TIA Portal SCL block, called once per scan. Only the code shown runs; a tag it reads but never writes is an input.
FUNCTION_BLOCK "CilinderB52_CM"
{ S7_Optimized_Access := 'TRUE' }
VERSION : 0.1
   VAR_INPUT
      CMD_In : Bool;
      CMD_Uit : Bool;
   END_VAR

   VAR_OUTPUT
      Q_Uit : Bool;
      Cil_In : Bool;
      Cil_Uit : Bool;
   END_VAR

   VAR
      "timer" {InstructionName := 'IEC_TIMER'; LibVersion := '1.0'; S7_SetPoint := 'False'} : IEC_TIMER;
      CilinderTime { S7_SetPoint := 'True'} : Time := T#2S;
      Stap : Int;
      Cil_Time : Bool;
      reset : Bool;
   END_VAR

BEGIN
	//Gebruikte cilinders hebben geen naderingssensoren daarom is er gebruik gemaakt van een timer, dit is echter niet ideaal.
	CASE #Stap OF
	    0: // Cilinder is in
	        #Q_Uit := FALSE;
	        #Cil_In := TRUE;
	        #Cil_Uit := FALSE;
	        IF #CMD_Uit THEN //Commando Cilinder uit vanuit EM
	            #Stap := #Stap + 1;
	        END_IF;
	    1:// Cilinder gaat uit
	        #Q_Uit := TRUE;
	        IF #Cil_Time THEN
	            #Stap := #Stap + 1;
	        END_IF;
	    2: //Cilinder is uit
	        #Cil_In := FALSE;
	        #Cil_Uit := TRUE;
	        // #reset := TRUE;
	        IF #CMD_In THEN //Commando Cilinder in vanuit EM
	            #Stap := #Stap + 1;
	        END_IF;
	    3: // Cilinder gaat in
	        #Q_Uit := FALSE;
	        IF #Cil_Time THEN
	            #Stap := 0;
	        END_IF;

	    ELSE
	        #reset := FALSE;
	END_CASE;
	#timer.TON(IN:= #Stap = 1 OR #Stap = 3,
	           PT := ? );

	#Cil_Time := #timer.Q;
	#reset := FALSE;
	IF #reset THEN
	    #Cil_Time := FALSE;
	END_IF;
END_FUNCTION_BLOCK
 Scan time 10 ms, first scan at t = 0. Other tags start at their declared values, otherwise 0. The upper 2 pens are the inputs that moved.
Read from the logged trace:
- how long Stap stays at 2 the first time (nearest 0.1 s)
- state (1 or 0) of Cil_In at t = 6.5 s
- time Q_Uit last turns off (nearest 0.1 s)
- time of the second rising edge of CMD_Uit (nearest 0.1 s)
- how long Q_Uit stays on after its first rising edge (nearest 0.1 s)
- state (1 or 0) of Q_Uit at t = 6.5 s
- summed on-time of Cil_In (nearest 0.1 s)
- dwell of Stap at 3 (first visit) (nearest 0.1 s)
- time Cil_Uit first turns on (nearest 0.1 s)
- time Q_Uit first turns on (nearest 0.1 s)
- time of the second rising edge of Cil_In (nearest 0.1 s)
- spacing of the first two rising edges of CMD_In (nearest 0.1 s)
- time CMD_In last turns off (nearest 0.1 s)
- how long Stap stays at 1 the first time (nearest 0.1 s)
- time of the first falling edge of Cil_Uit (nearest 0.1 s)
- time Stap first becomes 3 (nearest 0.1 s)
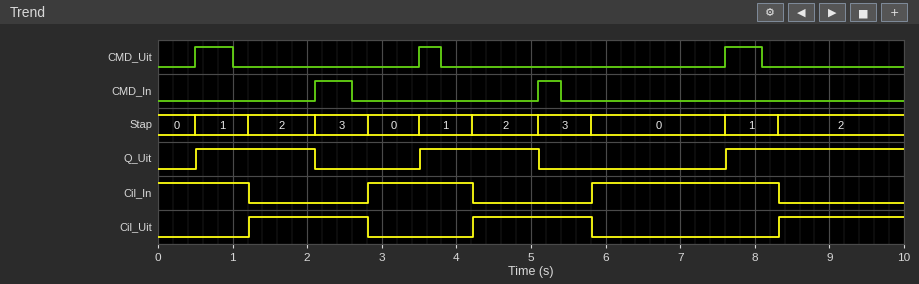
0.9 s
1
5.1 s
3.5 s
1.6 s
0
5.1 s
0.7 s
1.2 s
0.5 s
5.8 s
3.0 s
5.4 s
0.7 s
2.8 s
2.1 s
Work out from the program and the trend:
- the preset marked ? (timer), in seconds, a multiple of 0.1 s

0.7 s
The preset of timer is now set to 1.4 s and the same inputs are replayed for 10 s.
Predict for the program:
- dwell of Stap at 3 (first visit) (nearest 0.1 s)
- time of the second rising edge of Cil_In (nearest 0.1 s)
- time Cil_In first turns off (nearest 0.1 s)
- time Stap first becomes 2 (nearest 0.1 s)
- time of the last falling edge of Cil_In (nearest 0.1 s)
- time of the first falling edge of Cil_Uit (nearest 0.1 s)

1.4 s
6.5 s
1.9 s
1.9 s
9.0 s
3.5 s
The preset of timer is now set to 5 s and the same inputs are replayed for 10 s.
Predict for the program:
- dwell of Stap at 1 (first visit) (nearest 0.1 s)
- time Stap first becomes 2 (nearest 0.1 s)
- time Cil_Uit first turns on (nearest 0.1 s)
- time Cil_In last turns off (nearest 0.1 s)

5.0 s
5.5 s
5.5 s
5.5 s
